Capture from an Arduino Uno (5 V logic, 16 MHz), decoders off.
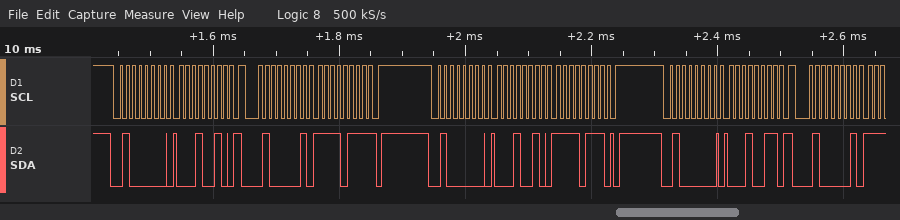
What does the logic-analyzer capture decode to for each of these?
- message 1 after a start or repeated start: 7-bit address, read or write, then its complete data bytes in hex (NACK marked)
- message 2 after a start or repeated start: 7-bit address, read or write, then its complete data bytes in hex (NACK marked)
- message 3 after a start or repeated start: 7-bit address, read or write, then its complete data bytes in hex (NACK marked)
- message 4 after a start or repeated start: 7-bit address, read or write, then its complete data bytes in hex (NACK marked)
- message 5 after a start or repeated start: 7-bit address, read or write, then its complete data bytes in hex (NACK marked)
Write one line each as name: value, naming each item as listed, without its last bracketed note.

message 1 after a start or repeated start: 7-bit address, read or write, then its complete data bytes in hex: 0x20 write: 12
message 2 after a start or repeated start: 7-bit address, read or write, then its complete data bytes in hex: 0x20 read: F7 NACK
message 3 after a start or repeated start: 7-bit address, read or write, then its complete data bytes in hex: 0x20 write: 12 F7
message 4 after a start or repeated start: 7-bit address, read or write, then its complete data bytes in hex: 0x20 write: 13
message 5 after a start or repeated start: 7-bit address, read or write, then its complete data bytes in hex: 0x20 read
